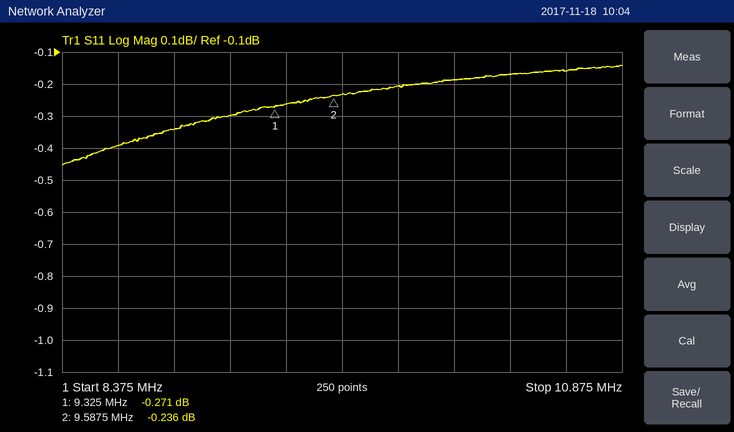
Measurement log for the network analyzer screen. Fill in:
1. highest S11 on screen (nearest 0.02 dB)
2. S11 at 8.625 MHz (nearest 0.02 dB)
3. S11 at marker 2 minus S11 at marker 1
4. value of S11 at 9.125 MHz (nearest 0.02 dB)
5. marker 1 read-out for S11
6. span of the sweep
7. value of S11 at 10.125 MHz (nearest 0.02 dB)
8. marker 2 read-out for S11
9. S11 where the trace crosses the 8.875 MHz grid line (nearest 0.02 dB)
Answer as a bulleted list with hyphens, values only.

- -0.14 dB
- -0.40 dB
- 0.035 dB
- -0.30 dB
- -0.271 dB
- 2.5 MHz
- -0.18 dB
- -0.236 dB
- -0.34 dB
